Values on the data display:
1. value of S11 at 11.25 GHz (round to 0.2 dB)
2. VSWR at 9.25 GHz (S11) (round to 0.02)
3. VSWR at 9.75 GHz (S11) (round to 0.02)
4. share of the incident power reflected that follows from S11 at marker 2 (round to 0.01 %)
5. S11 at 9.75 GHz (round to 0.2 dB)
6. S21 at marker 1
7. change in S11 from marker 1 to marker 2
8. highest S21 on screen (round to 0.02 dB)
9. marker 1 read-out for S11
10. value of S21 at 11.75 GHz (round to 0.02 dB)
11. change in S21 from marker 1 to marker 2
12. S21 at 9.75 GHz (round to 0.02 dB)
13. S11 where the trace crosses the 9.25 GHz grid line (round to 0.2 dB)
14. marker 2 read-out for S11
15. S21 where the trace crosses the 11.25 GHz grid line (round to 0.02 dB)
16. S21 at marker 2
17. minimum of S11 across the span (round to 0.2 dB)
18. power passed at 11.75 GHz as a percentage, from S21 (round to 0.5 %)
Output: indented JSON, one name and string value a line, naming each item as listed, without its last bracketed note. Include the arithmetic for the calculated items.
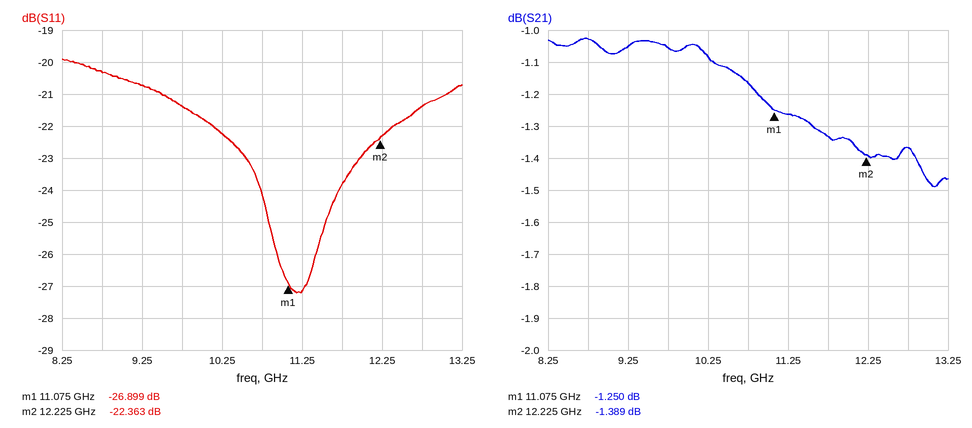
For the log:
{
  "value of S11 at 11.25 GHz": "-27.2 dB",
  "VSWR at 9.25 GHz (S11)": "|Γ| = 10^(-20.8/20) = 0.0912; VSWR = (1 + 0.0912)/(1 − 0.0912) ≈ 1.20",
  "VSWR at 9.75 GHz (S11)": "|Γ| = 10^(-21.4/20) = 0.0851; VSWR = (1 + 0.0851)/(1 − 0.0851) ≈ 1.19, so 1.18 to the nearest 0.02",
  "share of the incident power reflected that follows from S11 at marker 2": "10^(-22.363/10) ≈ 0.58 %",
  "S11 at 9.75 GHz": "-21.4 dB",
  "S21 at marker 1": "-1.250 dB",
  "change in S11 from marker 1 to marker 2": "-22.363 − (-26.899) = 4.536 dB",
  "highest S21 on screen": "-1.02 dB",
  "marker 1 read-out for S11": "-26.899 dB",
  "value of S21 at 11.75 GHz": "-1.34 dB",
  "change in S21 from marker 1 to marker 2": "-1.389 − (-1.25) = -0.139 dB",
  "S21 at 9.75 GHz": "-1.06 dB",
  "S11 where the trace crosses the 9.25 GHz grid line": "-20.8 dB",
  "marker 2 read-out for S11": "-22.363 dB",
  "S21 where the trace crosses the 11.25 GHz grid line": "-1.26 dB",
  "S21 at marker 2": "-1.389 dB",
  "minimum of S11 across the span": "-27.2 dB",
  "power passed at 11.75 GHz as a percentage, from S21": "10^(-1.34/10) ≈ 73.5 %"
}
